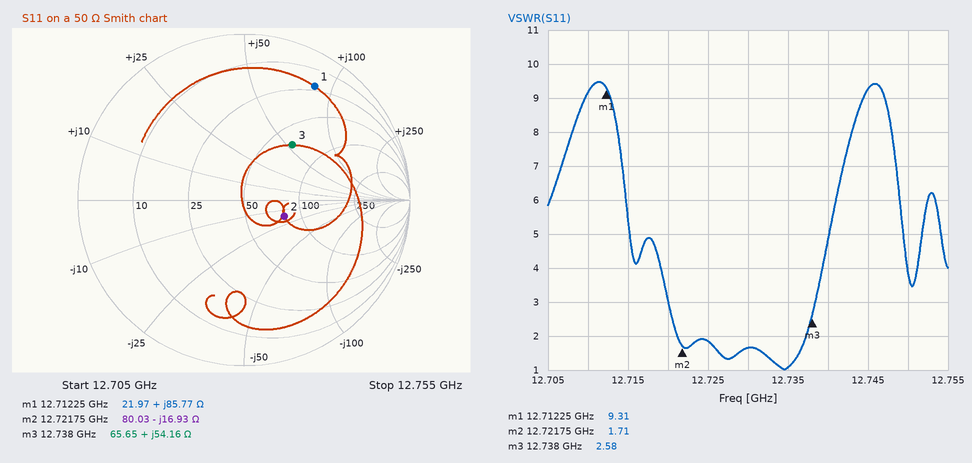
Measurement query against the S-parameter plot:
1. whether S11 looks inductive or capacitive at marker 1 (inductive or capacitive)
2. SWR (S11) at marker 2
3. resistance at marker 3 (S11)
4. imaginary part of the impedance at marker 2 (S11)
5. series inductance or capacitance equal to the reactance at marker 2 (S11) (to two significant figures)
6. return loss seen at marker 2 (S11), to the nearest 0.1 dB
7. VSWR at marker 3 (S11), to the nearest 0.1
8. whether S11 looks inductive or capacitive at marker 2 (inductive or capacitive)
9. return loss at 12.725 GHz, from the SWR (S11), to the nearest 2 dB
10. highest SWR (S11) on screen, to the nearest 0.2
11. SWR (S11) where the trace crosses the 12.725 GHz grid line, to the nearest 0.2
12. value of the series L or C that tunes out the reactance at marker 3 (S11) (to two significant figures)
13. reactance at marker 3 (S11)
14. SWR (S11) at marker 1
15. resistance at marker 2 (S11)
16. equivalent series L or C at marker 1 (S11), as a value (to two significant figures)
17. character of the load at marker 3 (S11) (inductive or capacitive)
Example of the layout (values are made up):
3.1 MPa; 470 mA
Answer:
inductive; 1.71; 65.65 Ω; -16.93 Ω; 740 fF; 11.6 dB; 2.6; capacitive; 10 dB; 9.4; 1.8; 230 fF; +54.16 Ω; 9.31; 80.03 Ω; 1.1 nH; inductive
